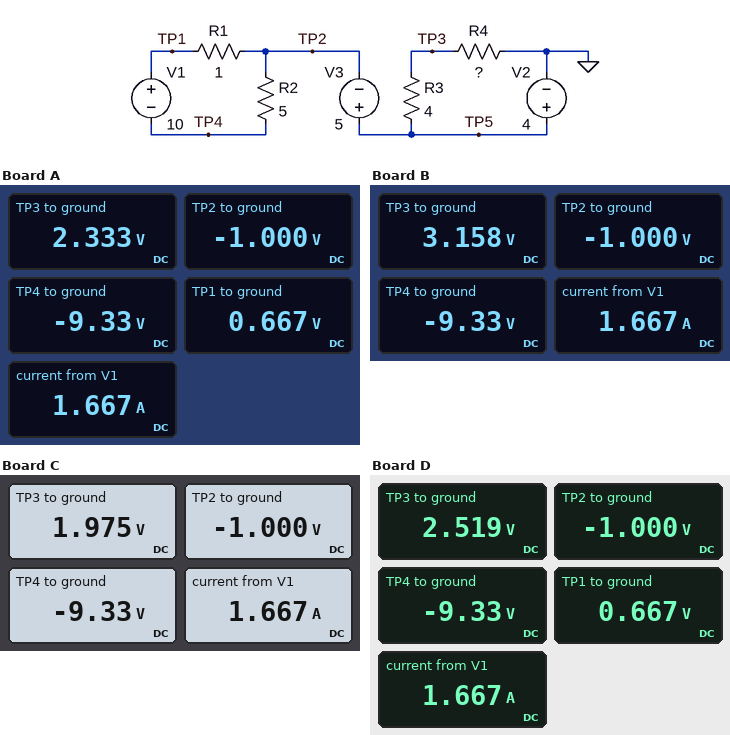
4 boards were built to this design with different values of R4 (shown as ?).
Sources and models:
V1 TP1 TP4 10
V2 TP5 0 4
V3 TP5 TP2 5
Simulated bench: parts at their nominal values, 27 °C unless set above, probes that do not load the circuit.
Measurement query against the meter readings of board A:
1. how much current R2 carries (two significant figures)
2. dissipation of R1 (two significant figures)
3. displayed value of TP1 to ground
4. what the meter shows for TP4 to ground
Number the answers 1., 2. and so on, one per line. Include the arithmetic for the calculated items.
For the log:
1. (-1 V - (-9.33 V)) / 5 Ω = 1.7 A
2. (667 mV - (-1 V))^2 / 1 Ω = 2.8 W
3. 0.667 V
4. -9.33 V
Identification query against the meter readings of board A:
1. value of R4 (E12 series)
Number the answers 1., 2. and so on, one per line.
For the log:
1. 5.6 Ω
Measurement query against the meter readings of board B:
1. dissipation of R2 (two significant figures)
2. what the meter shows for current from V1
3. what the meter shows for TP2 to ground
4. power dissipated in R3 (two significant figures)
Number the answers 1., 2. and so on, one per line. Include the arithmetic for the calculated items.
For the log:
1. (-1 V - (-9.33 V))^2 / 5 Ω = 14 W
2. 1.667 A
3. -1.000 V
4. (4 V - 3.158 V)^2 / 4 Ω = 180 mW
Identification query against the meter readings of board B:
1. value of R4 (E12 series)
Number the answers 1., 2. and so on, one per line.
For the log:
1. 15 Ω
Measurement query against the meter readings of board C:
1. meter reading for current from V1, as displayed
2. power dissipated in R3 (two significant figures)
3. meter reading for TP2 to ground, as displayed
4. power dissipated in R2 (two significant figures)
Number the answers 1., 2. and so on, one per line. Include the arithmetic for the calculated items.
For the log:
1. 1.667 A
2. (4 V - 1.975 V)^2 / 4 Ω = 1.0 W
3. -1.000 V
4. (-1 V - (-9.33 V))^2 / 5 Ω = 14 W
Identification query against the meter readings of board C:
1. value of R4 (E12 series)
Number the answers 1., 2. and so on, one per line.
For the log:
1. 3.9 Ω
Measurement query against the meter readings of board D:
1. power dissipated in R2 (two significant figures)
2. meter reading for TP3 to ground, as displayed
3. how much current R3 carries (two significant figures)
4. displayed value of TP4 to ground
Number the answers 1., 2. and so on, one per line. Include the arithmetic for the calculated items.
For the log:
1. (-1 V - (-9.33 V))^2 / 5 Ω = 14 W
2. 2.519 V
3. (4 V - 2.519 V) / 4 Ω = 370 mA
4. -9.33 V
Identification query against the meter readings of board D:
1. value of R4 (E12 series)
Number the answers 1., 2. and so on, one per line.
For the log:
1. 6.8 Ω
